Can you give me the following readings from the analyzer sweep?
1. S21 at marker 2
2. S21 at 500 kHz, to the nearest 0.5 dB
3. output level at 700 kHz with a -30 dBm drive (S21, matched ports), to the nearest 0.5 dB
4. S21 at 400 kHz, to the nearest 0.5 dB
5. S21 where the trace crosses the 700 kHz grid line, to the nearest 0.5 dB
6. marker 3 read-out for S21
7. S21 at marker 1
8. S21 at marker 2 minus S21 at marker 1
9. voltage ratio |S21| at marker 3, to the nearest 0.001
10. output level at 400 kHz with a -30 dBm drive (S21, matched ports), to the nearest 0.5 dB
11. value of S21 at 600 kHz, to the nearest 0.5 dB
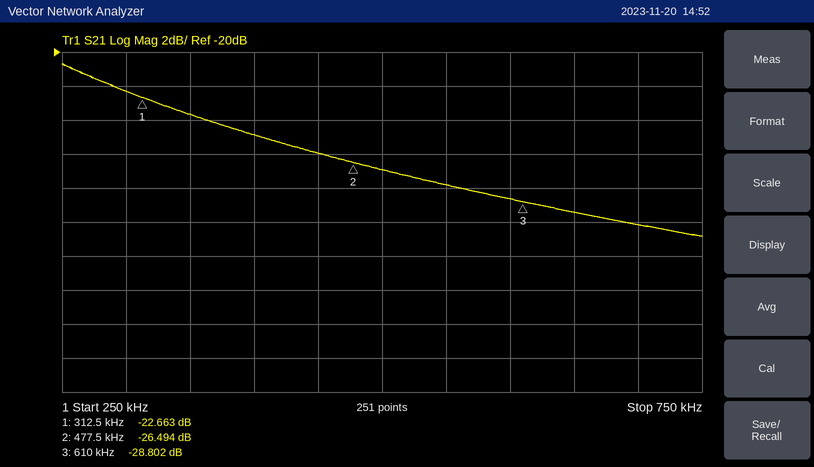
-26.494 dB
-27.0 dB
-60.0 dBm
-25.0 dB
-30.0 dB
-28.802 dB
-22.663 dB
-3.831 dB
0.036
-55.0 dBm
-28.5 dB
